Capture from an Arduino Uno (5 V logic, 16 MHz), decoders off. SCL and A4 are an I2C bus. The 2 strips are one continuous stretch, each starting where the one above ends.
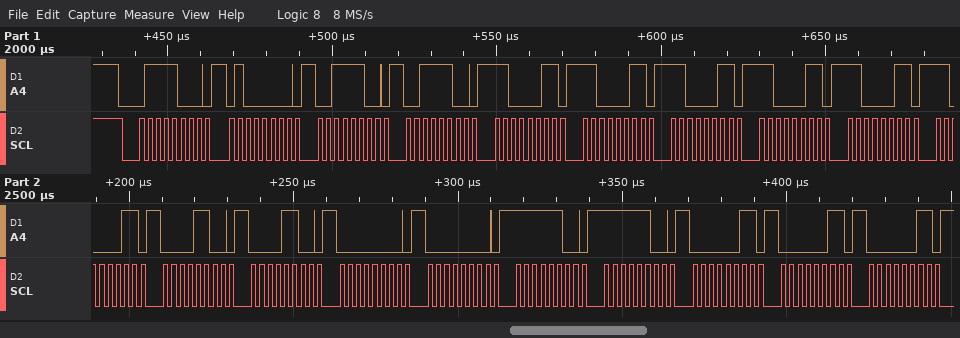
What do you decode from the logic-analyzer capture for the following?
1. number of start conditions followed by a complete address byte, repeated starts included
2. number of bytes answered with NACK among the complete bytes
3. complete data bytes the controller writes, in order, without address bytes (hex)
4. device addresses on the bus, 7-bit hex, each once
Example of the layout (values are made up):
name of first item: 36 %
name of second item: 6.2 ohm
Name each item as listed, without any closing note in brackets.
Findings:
number of start conditions followed by a complete address byte, repeated starts included: 1
number of bytes answered with NACK among the complete bytes: 0
complete data bytes the controller writes, in order, without address bytes: 40 3C 3C C3 C3 C3 C3 C3 C3 0C 0C 00 00 FC FC 03 03 03
device addresses on the bus, 7-bit hex, each once: 0x3C
